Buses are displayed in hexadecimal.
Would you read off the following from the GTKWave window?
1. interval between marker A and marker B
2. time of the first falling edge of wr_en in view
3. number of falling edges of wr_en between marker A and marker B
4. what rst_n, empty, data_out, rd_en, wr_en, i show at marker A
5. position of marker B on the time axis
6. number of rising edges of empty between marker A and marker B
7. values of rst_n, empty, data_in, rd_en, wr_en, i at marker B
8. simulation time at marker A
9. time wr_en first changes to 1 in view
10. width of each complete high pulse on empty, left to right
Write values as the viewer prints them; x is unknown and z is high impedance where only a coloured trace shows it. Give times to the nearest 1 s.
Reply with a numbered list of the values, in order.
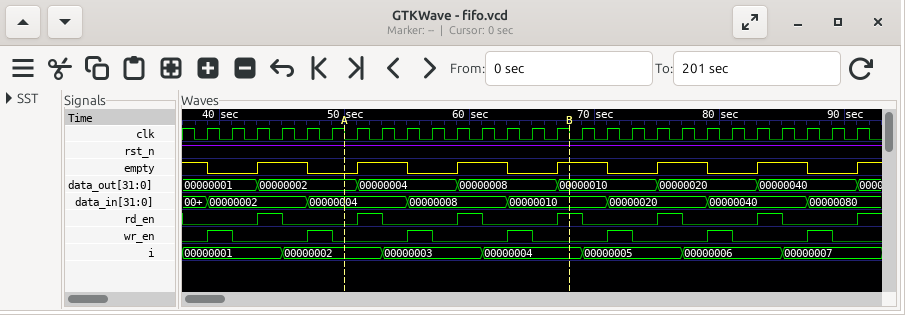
1. 18 s
2. 41 s
3. 2
4. rst_n=1, empty=0, data_out=00000002, rd_en=0, wr_en=0, i=00000002
5. 68 s
6. 3
7. rst_n=1, empty=1, data_in=00000010, rd_en=1, wr_en=0, i=00000004
8. 50 s
9. 39 s
10. 4 s, 4 s, 4 s, 4 s, 4 s, 4 s
